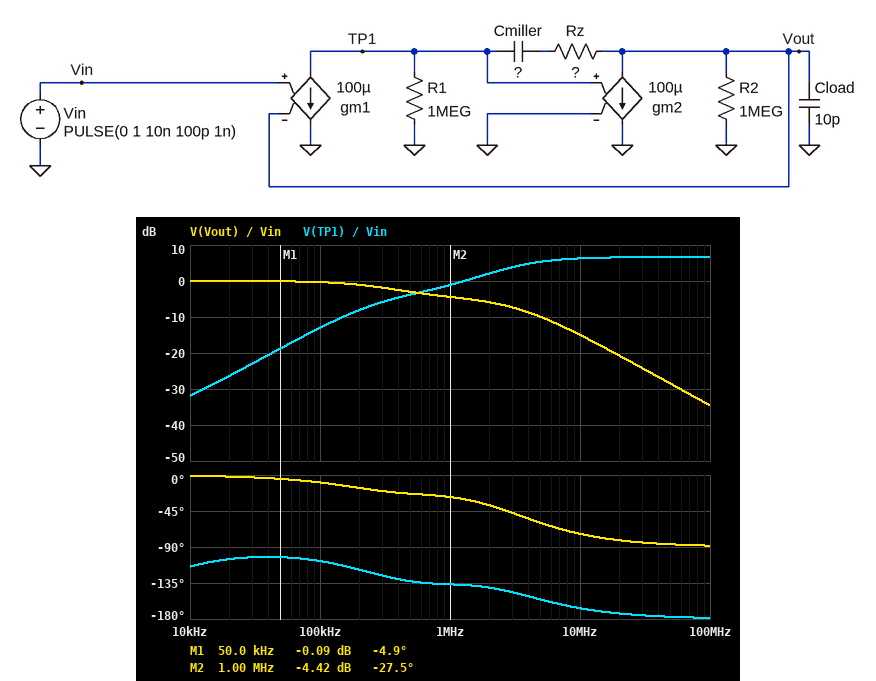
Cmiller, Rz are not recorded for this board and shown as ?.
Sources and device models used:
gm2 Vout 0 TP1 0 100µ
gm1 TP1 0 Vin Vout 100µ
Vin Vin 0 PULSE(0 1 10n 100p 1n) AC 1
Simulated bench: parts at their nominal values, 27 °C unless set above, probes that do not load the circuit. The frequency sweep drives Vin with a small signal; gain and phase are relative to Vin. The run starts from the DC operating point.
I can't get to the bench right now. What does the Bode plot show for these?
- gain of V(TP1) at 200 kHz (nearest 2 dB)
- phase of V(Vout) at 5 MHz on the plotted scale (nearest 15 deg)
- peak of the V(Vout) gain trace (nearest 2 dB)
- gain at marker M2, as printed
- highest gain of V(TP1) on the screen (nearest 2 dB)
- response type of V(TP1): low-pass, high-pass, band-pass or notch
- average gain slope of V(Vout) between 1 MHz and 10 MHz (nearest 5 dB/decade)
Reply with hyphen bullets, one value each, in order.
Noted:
- -8 dB
- -60 deg
- 0 dB
- -4.42 dB
- 6 dB
- high-pass
- -10 dB/decade
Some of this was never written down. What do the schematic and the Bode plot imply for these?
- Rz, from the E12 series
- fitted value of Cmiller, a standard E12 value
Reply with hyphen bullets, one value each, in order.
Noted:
- 22 kΩ
- 27 pF
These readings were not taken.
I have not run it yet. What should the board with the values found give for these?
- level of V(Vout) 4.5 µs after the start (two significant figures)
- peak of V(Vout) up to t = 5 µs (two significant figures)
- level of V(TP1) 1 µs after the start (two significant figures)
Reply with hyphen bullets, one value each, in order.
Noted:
- 1.0 V
- 1.0 V
- -97 mV
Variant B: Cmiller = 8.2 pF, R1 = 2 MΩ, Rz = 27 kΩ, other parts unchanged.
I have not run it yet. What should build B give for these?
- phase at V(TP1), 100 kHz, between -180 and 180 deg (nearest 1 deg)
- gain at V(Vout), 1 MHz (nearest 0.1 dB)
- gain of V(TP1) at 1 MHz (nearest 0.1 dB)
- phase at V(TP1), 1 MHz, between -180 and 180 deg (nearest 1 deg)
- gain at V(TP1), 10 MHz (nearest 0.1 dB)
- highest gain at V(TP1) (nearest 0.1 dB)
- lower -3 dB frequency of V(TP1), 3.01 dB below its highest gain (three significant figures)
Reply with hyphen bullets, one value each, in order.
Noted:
- -99 deg
- -1.4 dB
- -0.6 dB
- -118 deg
- 8.1 dB
- 8.5 dB
- 3.11 MHz
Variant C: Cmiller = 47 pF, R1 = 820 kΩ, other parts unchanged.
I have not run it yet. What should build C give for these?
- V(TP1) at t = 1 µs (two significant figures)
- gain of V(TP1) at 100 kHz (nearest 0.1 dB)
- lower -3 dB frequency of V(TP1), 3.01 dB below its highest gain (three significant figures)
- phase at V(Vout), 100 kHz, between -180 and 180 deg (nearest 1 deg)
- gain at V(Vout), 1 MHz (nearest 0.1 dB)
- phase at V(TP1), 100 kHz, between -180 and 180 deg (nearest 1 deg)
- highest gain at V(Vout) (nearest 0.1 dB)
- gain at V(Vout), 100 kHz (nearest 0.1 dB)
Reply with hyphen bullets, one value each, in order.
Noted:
- -190 mV
- -10.2 dB
- 3.05 MHz
- -14 deg
- -5.1 dB
- -119 deg
- 0 dB
- -0.9 dB
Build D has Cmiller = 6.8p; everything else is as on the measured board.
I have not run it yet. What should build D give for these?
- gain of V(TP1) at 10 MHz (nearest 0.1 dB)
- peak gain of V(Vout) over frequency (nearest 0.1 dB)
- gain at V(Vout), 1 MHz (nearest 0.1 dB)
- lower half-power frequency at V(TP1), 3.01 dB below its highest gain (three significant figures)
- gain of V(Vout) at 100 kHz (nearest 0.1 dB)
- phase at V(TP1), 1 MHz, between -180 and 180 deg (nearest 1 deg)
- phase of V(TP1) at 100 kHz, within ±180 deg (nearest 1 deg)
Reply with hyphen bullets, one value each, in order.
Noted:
- 6.6 dB
- 0 dB
- -0.6 dB
- 1.71 MHz
- 0 dB
- -114 deg
- -98 deg
